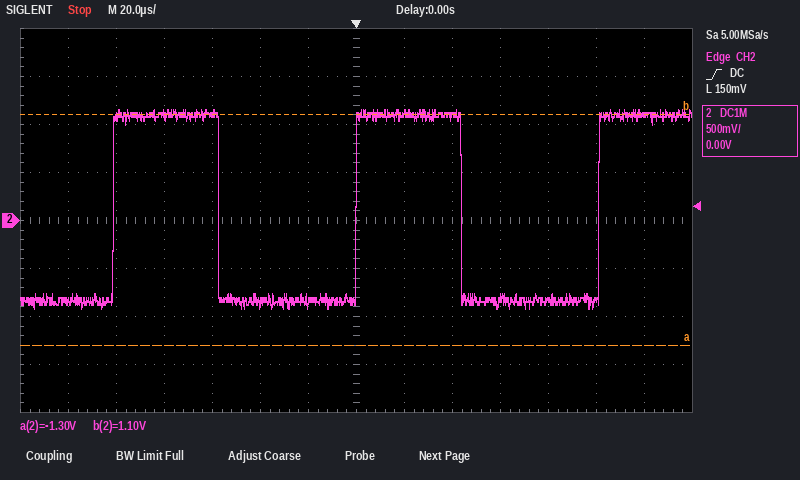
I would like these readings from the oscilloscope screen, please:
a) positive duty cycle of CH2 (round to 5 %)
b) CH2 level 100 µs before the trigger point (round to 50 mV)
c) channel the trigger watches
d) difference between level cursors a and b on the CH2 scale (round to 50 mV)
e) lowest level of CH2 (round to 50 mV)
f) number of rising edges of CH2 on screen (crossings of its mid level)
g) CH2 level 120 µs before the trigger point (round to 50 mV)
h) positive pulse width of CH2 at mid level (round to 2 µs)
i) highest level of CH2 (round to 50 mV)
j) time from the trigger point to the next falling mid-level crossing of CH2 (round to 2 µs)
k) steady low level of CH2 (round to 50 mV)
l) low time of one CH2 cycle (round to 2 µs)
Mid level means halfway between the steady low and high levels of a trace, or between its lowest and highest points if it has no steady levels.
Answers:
45 %
1.10 V
CH2
2.40 V
-900 mV
3
-850 mV
44 µs
1.15 V
44 µs
-850 mV
58 µs
